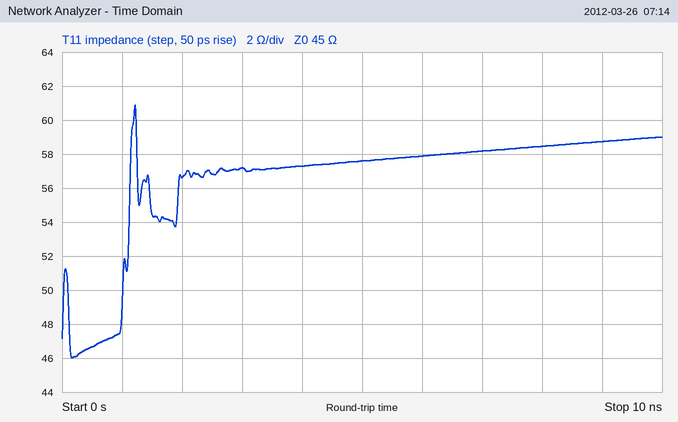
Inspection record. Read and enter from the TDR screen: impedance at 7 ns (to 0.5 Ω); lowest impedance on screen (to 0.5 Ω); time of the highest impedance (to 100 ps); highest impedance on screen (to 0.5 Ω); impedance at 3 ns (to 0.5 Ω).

58.0 Ω
46.0 Ω
1.2 ns
61.0 Ω
57.0 Ω
